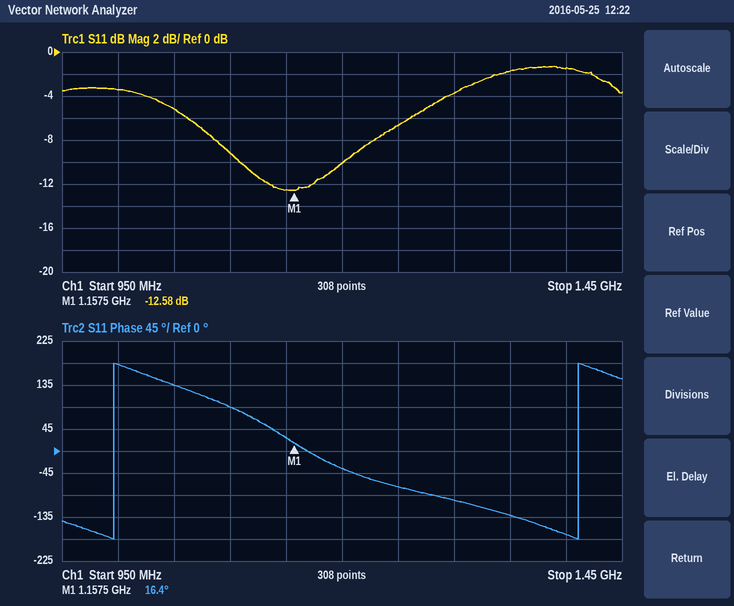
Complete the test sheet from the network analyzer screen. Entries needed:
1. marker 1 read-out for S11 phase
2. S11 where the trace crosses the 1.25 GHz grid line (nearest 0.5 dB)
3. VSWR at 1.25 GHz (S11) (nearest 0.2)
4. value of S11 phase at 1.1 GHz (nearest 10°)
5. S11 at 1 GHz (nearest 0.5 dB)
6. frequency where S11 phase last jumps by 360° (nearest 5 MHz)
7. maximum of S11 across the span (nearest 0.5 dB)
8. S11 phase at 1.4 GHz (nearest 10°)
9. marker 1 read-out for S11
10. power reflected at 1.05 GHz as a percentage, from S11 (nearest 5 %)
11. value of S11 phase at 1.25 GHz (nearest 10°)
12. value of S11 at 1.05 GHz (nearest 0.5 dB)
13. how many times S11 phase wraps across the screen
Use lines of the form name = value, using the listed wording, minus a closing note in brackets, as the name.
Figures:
marker 1 read-out for S11 phase = 16.4°
S11 where the trace crosses the 1.25 GHz grid line = -6.5 dB
VSWR at 1.25 GHz (S11) = 2.8
value of S11 phase at 1.1 GHz = 90°
S11 at 1 GHz = -3.5 dB
frequency where S11 phase last jumps by 360° = 1.410 GHz
maximum of S11 across the span = -1.5 dB
S11 phase at 1.4 GHz = -170°
marker 1 read-out for S11 = -12.58 dB
power reflected at 1.05 GHz as a percentage, from S11 = 30 %
value of S11 phase at 1.25 GHz = -70°
value of S11 at 1.05 GHz = -5.0 dB
how many times S11 phase wraps across the screen = 2
